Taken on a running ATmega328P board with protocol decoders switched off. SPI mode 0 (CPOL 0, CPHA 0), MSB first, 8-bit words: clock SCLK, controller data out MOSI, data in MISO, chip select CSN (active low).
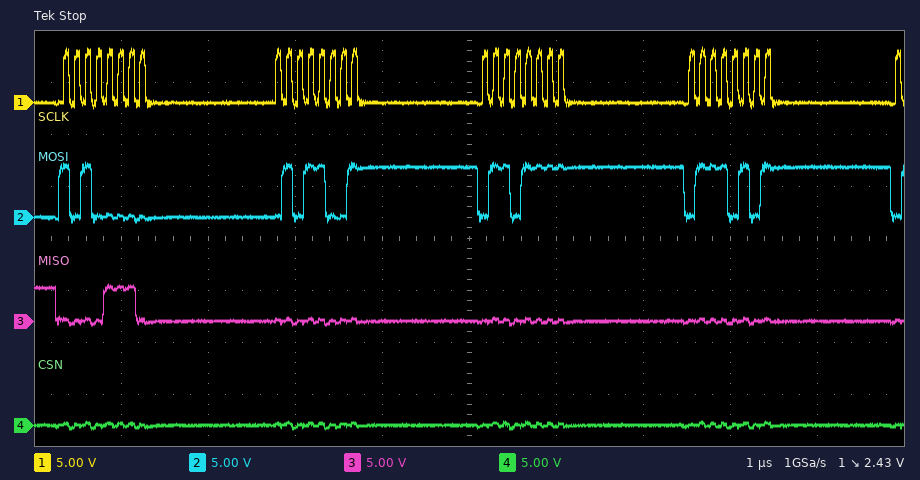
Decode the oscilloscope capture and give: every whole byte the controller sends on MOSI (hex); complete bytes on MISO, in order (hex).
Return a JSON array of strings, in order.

["A0 59 6F 75", "0E 00 00 00"]
